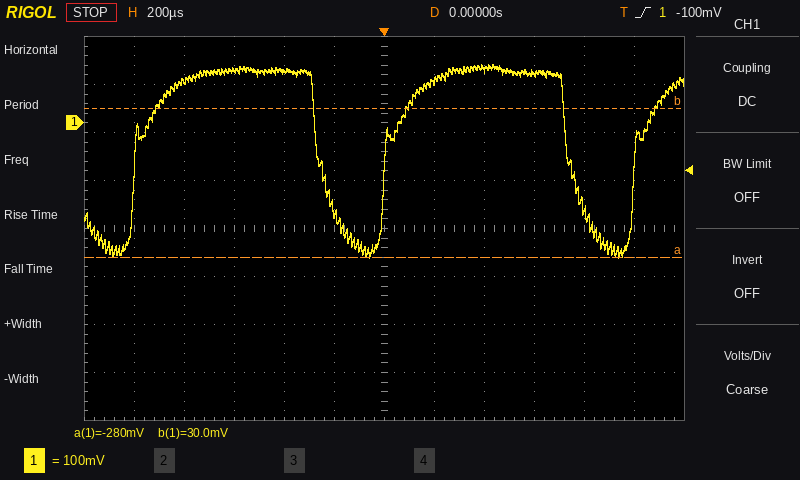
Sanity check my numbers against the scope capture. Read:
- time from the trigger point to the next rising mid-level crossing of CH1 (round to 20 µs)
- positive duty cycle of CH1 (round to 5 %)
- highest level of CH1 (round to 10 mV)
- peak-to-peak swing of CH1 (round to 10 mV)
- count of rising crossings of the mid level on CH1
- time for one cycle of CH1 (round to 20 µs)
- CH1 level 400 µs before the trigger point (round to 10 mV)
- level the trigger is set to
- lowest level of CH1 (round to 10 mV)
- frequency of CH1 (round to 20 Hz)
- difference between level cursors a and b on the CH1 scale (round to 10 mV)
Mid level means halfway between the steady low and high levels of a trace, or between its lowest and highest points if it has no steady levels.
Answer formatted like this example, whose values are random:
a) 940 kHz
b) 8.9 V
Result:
a) 1.00 ms
b) 75 %
c) 120 mV
d) 400 mV
e) 3
f) 1.00 ms
g) 110 mV
h) -100 mV
i) -280 mV
j) 1.00 kHz
k) 310 mV
